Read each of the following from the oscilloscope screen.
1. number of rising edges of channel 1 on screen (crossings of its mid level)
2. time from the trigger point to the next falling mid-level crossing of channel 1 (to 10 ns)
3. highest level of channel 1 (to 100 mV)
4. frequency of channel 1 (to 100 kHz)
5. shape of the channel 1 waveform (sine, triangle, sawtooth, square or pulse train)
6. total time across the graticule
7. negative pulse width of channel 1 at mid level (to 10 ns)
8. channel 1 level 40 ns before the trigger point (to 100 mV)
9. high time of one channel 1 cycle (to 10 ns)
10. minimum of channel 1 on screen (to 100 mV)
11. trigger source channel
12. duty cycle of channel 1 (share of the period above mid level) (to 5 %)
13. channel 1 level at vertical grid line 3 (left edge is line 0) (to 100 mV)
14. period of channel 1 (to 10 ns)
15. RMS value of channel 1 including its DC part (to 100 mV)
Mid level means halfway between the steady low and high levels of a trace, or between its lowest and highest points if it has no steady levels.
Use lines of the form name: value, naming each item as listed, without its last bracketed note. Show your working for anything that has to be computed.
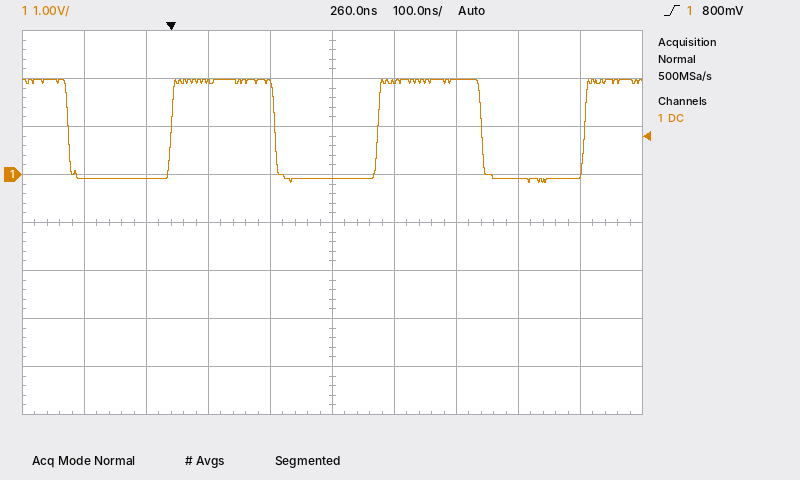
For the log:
number of rising edges of channel 1 on screen: 3
time from the trigger point to the next falling mid-level crossing of channel 1: 170 ns
highest level of channel 1: 2.0 V
frequency of channel 1: 1 / 330 ns ≈ 3.0 MHz
shape of the channel 1 waveform: square
total time across the graticule: 1 µs
negative pulse width of channel 1 at mid level: 170 ns
channel 1 level 40 ns before the trigger point: -100 mV
high time of one channel 1 cycle: 170 ns
minimum of channel 1 on screen: -200 mV
trigger source channel: channel 1
duty cycle of channel 1 (share of the period above mid level): 170 ns / 330 ns ≈ 51.5 %, so 50 % to the nearest 5 %
channel 1 level at vertical grid line 3 (left edge is line 0): 1.9 V
period of channel 1: 330 ns
RMS value of channel 1 including its DC part: √(0.5 × (2.0 V)² + 0.5 × (-200 mV)²) ≈ 1.4 V
